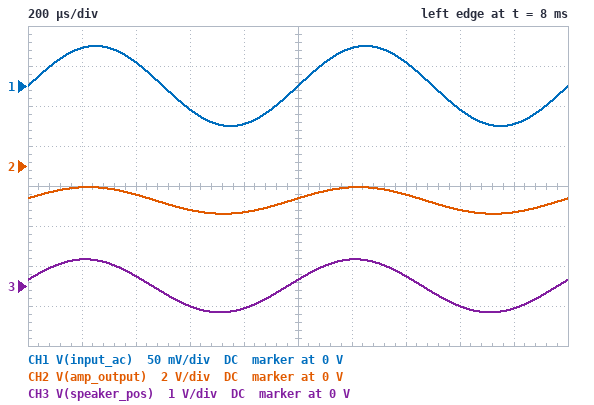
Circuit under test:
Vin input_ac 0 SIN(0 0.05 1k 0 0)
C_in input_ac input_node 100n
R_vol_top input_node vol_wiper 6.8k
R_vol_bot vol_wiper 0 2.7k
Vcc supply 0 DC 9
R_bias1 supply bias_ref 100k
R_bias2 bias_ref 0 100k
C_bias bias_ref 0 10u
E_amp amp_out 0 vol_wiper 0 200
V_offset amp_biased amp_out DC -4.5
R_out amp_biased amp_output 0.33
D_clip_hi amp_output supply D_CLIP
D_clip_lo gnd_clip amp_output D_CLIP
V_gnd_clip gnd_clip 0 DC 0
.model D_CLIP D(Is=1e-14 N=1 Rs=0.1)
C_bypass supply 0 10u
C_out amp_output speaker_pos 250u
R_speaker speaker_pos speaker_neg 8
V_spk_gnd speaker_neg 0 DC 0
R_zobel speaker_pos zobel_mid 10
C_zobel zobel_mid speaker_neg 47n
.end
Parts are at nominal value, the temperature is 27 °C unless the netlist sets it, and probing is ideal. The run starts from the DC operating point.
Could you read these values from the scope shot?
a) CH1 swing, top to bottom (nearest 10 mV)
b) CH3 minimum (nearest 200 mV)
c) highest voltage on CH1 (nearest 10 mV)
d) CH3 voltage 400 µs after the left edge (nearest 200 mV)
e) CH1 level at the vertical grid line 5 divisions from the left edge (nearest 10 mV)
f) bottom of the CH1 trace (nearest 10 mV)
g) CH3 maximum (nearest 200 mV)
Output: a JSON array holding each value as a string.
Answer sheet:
["100 mV", "-600 mV", "50 mV", "200 mV", "0 V", "-50 mV", "600 mV"]
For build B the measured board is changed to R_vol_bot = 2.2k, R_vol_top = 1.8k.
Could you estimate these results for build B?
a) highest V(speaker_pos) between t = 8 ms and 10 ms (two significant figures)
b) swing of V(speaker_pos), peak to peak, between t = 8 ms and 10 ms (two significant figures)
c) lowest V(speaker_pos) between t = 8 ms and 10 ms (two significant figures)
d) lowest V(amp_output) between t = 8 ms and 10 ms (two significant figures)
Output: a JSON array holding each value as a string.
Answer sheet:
["2.1 V", "3.4 V", "-1.4 V", "-2.9 V"]
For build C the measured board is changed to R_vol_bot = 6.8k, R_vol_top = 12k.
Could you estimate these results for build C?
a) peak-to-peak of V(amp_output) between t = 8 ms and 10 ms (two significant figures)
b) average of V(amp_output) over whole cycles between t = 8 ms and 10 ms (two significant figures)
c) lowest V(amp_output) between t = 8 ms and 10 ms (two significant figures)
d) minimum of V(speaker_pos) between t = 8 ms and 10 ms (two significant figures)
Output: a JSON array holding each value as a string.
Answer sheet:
["1.7 V", "-1.7 V", "-2.6 V", "-850 mV"]
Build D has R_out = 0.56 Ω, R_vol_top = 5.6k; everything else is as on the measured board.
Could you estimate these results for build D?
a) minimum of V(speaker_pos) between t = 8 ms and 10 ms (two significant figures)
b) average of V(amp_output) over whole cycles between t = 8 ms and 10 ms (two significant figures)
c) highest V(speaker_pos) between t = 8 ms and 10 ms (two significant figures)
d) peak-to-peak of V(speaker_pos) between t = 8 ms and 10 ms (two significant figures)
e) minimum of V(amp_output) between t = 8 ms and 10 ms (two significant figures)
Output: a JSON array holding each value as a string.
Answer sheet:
["-500 mV", "-1.4 V", "510 mV", "1.0 V", "-1.9 V"]
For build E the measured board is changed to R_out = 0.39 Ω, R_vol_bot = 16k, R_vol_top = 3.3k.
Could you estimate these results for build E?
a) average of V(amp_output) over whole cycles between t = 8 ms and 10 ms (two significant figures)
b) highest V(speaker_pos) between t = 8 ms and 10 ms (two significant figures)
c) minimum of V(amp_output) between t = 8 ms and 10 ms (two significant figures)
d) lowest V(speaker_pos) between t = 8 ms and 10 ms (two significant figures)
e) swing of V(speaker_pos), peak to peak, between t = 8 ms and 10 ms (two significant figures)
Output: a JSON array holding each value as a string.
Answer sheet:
["-810 mV", "4.4 V", "-3.3 V", "-2.5 V", "6.8 V"]
